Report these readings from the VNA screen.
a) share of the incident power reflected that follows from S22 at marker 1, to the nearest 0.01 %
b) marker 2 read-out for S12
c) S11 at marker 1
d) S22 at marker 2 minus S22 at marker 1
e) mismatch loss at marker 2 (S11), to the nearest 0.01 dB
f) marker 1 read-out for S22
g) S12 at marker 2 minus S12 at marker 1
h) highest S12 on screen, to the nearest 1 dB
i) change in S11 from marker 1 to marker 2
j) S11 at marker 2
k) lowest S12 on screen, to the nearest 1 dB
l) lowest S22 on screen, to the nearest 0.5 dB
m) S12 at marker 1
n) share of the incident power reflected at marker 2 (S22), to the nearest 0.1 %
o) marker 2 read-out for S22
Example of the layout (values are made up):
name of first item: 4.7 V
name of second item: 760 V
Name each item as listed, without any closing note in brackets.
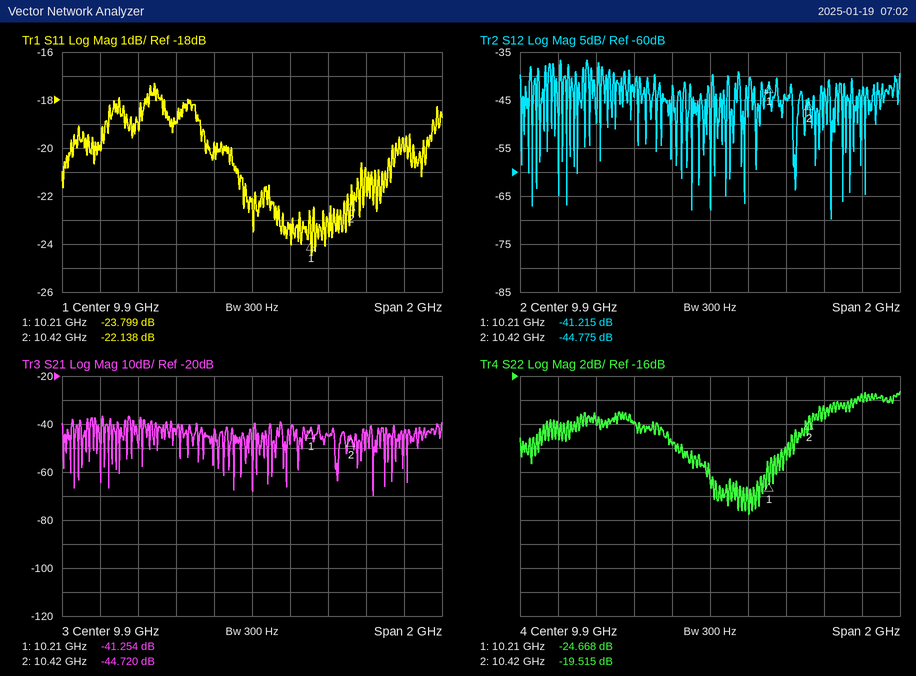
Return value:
share of the incident power reflected that follows from S22 at marker 1, to the nearest 0.01 %: 0.34 %
marker 2 read-out for S12: -44.775 dB
S11 at marker 1: -23.799 dB
S22 at marker 2 minus S22 at marker 1: 5.153 dB
mismatch loss at marker 2 (S11), to the nearest 0.01 dB: 0.03 dB
marker 1 read-out for S22: -24.668 dB
S12 at marker 2 minus S12 at marker 1: -3.560 dB
highest S12 on screen, to the nearest 1 dB: -37 dB
change in S11 from marker 1 to marker 2: 1.661 dB
S11 at marker 2: -22.138 dB
lowest S12 on screen, to the nearest 1 dB: -70 dB
lowest S22 on screen, to the nearest 0.5 dB: -27.5 dB
S12 at marker 1: -41.215 dB
share of the incident power reflected at marker 2 (S22), to the nearest 0.1 %: 1.1 %
marker 2 read-out for S22: -19.515 dB
